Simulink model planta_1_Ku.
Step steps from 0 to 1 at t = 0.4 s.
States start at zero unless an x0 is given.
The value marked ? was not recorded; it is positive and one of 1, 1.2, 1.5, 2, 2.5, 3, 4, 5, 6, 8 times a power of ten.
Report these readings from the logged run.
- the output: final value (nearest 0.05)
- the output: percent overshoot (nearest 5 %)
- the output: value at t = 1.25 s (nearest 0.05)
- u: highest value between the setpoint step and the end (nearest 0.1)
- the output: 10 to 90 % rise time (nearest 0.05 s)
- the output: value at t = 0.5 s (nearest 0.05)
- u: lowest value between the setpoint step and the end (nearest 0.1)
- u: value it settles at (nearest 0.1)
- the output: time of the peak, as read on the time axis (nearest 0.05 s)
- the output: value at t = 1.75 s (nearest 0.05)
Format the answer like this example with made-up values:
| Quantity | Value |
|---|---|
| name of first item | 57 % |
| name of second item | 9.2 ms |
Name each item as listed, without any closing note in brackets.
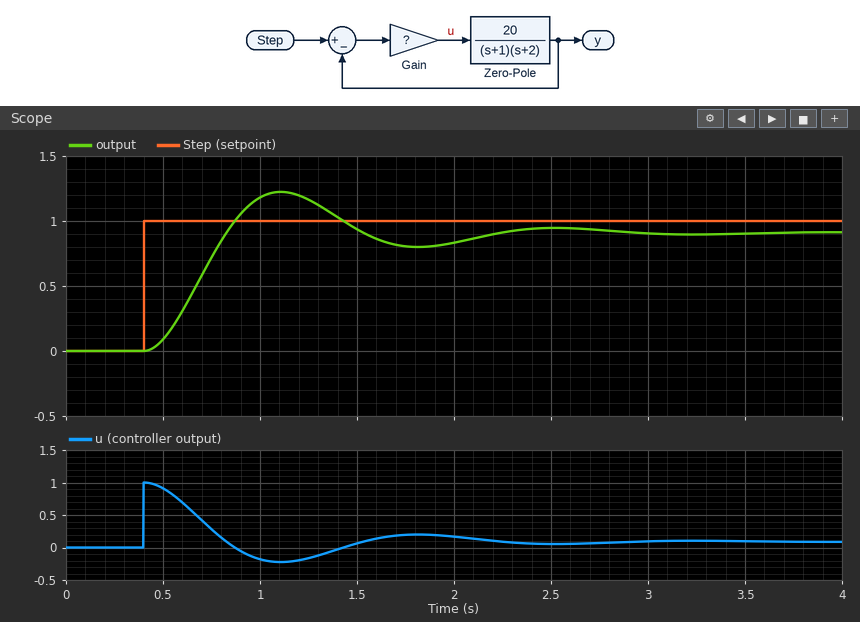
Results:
| Quantity | Value |
|---|---|
| the output: final value | 0.90 |
| the output: percent overshoot | 35 % |
| the output: value at t = 1.25 s | 1.15 |
| u: highest value between the setpoint step and the end | 1.0 |
| the output: 10 to 90 % rise time | 0.30 s |
| the output: value at t = 0.5 s | 0.10 |
| u: lowest value between the setpoint step and the end | -0.2 |
| u: value it settles at | 0.1 |
| the output: time of the peak, as read on the time axis | 1.10 s |
| the output: value at t = 1.75 s | 0.80 |
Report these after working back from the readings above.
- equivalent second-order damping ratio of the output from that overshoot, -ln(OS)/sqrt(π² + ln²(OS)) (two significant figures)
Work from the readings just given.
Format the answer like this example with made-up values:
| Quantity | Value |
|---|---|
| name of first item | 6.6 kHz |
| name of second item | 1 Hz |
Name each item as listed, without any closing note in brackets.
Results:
| Quantity | Value |
|---|---|
| equivalent second-order damping ratio of the output from that overshoot, -ln(OS)/sqrt(π² + ln²(OS)) | 0.32 |
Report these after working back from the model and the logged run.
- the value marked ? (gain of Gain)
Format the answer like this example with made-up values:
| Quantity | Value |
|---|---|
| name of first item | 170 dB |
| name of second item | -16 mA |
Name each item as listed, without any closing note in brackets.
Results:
| Quantity | Value |
|---|---|
| the value marked ? | 1 |
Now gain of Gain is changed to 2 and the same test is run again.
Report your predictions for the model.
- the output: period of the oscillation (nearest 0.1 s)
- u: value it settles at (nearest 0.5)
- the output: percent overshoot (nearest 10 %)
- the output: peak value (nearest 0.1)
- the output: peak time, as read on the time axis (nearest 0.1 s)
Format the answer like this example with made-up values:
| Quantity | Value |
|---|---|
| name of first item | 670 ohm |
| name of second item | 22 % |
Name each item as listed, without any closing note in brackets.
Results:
| Quantity | Value |
|---|---|
| the output: period of the oscillation | 1.0 s |
| u: value it settles at | 0.0 |
| the output: percent overshoot | 50 % |
| the output: peak value | 1.4 |
| the output: peak time, as read on the time axis | 0.9 s |
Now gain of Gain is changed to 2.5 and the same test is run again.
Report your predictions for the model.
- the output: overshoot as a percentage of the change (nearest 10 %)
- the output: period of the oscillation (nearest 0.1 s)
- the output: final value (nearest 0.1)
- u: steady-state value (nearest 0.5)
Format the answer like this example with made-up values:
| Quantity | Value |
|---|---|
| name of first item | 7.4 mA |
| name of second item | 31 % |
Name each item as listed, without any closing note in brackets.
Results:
| Quantity | Value |
|---|---|
| the output: overshoot as a percentage of the change | 50 % |
| the output: period of the oscillation | 0.9 s |
| the output: final value | 1.0 |
| u: steady-state value | 0.0 |
